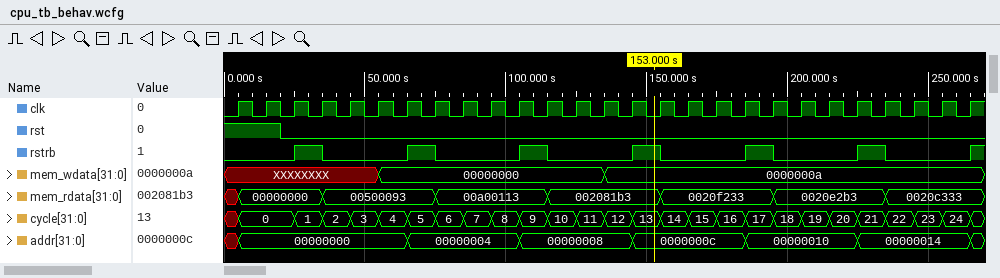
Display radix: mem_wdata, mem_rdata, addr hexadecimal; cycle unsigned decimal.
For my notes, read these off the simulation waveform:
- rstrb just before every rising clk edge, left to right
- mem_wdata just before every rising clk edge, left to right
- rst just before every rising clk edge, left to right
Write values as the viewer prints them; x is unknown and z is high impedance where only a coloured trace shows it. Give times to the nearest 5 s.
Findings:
0 0 0 1 0 0 0 1 0 0 0 1 0 0 0 1 0 0 0 1 0 0 0 1 0 0 0
XXXXXXXX, XXXXXXXX, XXXXXXXX, XXXXXXXX, XXXXXXXX, XXXXXXXX, 00000000, 00000000, 00000000, 00000000, 00000000, 00000000, 00000000, 00000000, 0000000a, 0000000a, 0000000a, 0000000a, 0000000a, 0000000a, 0000000a, 0000000a, 0000000a, 0000000a, 0000000a, 0000000a, 0000000a
1 1 0 0 0 0 0 0 0 0 0 0 0 0 0 0 0 0 0 0 0 0 0 0 0 0 0
